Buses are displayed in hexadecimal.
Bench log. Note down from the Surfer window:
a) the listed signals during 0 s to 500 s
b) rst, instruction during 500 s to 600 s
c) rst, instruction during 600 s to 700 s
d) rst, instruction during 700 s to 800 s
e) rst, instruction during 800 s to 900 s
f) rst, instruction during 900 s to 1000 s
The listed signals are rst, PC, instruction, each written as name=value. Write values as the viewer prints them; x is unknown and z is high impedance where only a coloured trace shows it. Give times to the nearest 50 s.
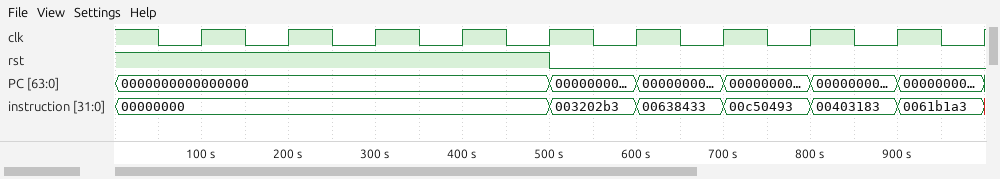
rst=1, PC=0000000000000000, instruction=00000000
rst=0, instruction=003202b3
rst=0, instruction=00638433
rst=0, instruction=00c50493
rst=0, instruction=00403183
rst=0, instruction=0061b1a3
